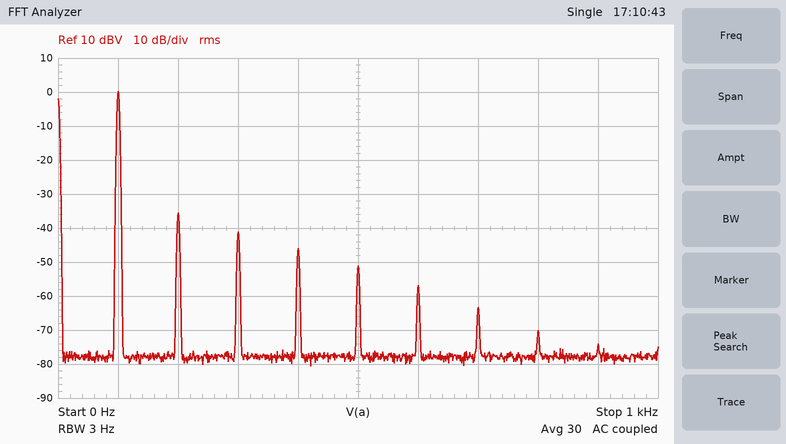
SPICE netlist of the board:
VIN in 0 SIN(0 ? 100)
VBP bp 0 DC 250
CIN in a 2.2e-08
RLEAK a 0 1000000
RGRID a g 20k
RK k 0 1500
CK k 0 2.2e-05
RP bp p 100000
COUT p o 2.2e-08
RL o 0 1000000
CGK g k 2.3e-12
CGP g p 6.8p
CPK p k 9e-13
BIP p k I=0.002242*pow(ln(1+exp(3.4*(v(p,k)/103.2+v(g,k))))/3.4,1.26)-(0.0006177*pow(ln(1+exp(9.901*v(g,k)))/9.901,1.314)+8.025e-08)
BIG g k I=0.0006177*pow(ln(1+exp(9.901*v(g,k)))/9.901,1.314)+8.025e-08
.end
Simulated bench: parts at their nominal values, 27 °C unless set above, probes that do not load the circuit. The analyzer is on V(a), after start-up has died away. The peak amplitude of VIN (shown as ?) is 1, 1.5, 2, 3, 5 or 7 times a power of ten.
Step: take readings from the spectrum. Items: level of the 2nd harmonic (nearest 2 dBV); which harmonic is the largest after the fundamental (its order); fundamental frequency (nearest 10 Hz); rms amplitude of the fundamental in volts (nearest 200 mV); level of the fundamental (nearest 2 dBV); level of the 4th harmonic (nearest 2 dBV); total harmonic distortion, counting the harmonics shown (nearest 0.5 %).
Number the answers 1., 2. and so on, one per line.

1. -36 dBV
2. 2
3. 100 Hz
4. 1.0 V
5. 0 dBV
6. -46 dBV
7. 2.0 %
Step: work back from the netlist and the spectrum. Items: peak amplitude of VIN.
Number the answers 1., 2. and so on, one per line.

1. 1.5 V
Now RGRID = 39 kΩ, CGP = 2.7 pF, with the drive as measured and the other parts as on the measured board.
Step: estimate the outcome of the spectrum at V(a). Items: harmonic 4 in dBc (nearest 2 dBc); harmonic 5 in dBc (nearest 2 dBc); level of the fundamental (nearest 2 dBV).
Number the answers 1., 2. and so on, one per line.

1. -48 dBc
2. -54 dBc
3. 0 dBV
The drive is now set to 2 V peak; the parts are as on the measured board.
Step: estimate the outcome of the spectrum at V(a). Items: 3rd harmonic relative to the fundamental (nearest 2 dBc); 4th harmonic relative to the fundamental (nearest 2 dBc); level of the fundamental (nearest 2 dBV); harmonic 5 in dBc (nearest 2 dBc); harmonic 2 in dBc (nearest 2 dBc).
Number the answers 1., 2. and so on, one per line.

1. -38 dBc
2. -42 dBc
3. 2 dBV
4. -48 dBc
5. -32 dBc
